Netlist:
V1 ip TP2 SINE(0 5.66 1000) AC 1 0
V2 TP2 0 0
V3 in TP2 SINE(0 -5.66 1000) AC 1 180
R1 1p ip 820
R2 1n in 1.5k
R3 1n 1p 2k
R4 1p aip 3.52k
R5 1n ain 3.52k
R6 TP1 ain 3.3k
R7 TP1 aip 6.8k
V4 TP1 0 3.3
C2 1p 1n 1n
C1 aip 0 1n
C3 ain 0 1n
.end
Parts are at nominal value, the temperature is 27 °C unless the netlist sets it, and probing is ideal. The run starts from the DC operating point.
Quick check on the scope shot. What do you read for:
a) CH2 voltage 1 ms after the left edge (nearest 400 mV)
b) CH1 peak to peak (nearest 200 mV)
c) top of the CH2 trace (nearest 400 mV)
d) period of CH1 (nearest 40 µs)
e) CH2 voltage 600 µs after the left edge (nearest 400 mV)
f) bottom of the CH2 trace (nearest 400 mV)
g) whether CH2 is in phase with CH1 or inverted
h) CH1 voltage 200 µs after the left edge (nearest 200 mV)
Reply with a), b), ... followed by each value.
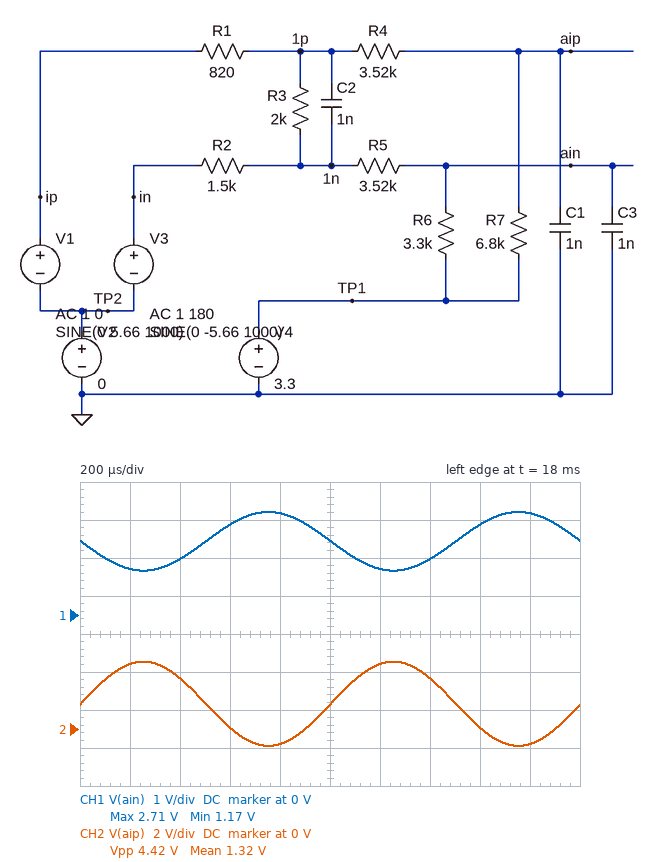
a) 1.2 V
b) 1.6 V
c) 3.6 V
d) 1.00 ms
e) 0 V
f) -800 mV
g) inverted
h) 1.2 V
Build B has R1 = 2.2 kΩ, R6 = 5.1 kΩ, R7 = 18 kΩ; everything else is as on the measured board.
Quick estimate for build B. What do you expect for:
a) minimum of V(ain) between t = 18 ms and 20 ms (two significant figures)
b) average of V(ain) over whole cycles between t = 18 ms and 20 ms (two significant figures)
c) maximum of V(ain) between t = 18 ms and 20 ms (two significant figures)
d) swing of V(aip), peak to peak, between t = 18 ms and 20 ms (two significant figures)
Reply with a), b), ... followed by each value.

a) 190 mV
b) 1.6 V
c) 3.0 V
d) 2.3 V
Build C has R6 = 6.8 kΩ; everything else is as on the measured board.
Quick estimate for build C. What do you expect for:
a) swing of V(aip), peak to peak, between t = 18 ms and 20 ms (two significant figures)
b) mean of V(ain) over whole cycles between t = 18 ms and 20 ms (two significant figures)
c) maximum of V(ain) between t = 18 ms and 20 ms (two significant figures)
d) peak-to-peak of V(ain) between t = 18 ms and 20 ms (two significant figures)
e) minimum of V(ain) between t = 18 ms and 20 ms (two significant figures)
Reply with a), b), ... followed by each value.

a) 4.4 V
b) 1.4 V
c) 2.5 V
d) 2.2 V
e) 270 mV
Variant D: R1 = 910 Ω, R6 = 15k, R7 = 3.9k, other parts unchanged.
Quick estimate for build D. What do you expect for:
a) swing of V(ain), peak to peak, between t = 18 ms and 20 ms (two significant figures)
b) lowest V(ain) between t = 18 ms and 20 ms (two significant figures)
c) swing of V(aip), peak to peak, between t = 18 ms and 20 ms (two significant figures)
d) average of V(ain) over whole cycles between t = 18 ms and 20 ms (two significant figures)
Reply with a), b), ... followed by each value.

a) 3.0 V
b) -630 mV
c) 3.2 V
d) 860 mV
